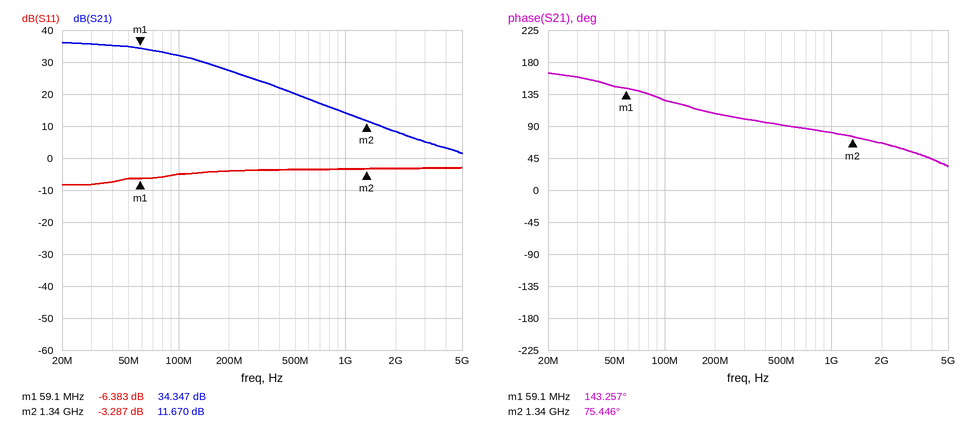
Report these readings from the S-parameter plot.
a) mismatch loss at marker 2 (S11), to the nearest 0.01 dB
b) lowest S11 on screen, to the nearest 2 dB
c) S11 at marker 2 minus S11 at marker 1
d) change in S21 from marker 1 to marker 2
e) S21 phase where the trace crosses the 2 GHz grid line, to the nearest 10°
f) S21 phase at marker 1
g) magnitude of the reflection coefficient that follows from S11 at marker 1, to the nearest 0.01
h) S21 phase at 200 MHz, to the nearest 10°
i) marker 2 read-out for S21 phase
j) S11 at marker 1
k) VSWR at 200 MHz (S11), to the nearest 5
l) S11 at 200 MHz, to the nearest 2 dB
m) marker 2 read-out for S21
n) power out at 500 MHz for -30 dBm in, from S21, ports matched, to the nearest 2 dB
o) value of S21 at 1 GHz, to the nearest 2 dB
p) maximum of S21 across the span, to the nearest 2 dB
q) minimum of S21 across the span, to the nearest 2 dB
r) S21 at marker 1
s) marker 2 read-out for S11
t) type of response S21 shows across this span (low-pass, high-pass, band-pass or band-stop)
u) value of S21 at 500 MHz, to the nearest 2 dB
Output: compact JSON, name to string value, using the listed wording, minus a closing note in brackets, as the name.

{"mismatch loss at marker 2 (S11), to the nearest 0.01 dB": "2.75 dB", "lowest S11 on screen, to the nearest 2 dB": "-8 dB", "S11 at marker 2 minus S11 at marker 1": "3.096 dB", "change in S21 from marker 1 to marker 2": "-22.677 dB", "S21 phase where the trace crosses the 2 GHz grid line, to the nearest 10°": "70°", "S21 phase at marker 1": "143.257°", "magnitude of the reflection coefficient that follows from S11 at marker 1, to the nearest 0.01": "0.48", "S21 phase at 200 MHz, to the nearest 10°": "110°", "marker 2 read-out for S21 phase": "75.446°", "S11 at marker 1": "-6.383 dB", "VSWR at 200 MHz (S11), to the nearest 5": "5", "S11 at 200 MHz, to the nearest 2 dB": "-4 dB", "marker 2 read-out for S21": "11.670 dB", "power out at 500 MHz for -30 dBm in, from S21, ports matched, to the nearest 2 dB": "-10 dBm", "value of S21 at 1 GHz, to the nearest 2 dB": "14 dB", "maximum of S21 across the span, to the nearest 2 dB": "36 dB", "minimum of S21 across the span, to the nearest 2 dB": "2 dB", "S21 at marker 1": "34.347 dB", "marker 2 read-out for S11": "-3.287 dB", "type of response S21 shows across this span": "low-pass", "value of S21 at 500 MHz, to the nearest 2 dB": "20 dB"}
